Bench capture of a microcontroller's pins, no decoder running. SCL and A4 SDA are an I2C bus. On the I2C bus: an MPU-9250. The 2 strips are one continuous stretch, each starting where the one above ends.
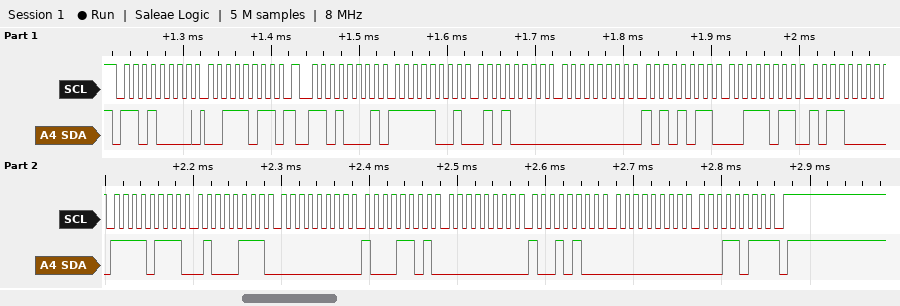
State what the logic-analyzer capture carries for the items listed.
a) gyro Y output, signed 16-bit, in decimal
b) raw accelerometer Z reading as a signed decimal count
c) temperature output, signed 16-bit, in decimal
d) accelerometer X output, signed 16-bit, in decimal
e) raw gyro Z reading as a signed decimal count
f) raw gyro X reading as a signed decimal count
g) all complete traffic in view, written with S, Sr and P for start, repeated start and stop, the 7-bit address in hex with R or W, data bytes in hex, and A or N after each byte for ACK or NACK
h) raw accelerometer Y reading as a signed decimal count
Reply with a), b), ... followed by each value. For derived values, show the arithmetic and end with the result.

a) 0x0094 = 148
b) 0x3BB0 = 15280
c) 0xF747 = -2233
d) 0xF950 = -1712
e) 0x001B = 27
f) 0x008D = 141
g) S 68W A 3B A Sr 68R A F9 A 50 A 00 A AB A 3B A B0 A F7 A 47 A 00 A 8D A 00 A 94 A 00 A 1B N P
h) 0x00AB = 171
